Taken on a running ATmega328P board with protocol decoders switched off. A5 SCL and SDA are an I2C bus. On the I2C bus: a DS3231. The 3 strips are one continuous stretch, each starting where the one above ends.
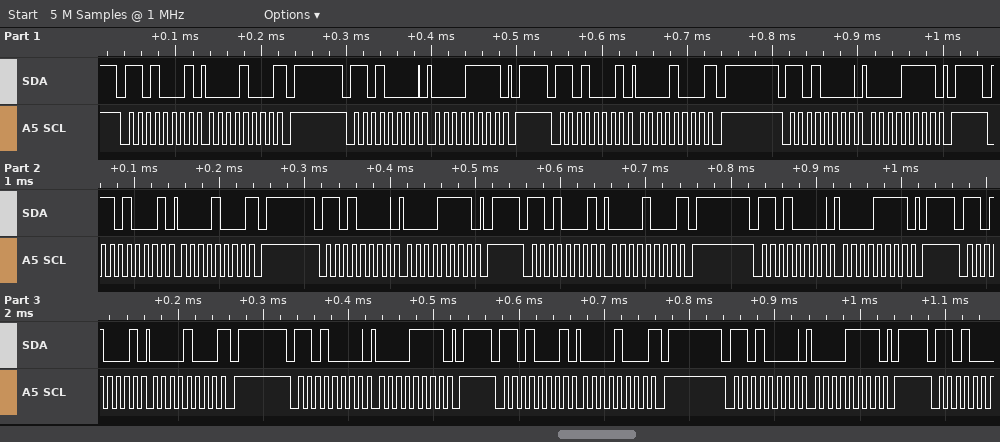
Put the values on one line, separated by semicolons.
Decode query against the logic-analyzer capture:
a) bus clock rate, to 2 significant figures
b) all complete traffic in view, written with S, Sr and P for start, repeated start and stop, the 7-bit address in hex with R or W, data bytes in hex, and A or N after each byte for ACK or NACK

100 kHz; S 68R A 08 N P S 68W A 0F A P S 68R A 08 N P S 68W A 0F A P S 68R A 08 N P S 68W A 0F A P S 68R A 08 N P S 68W A 0F A P S 68R A 08 N P S 68W A 0F A P S 68R A 08 N P S 68W A 0F A P
